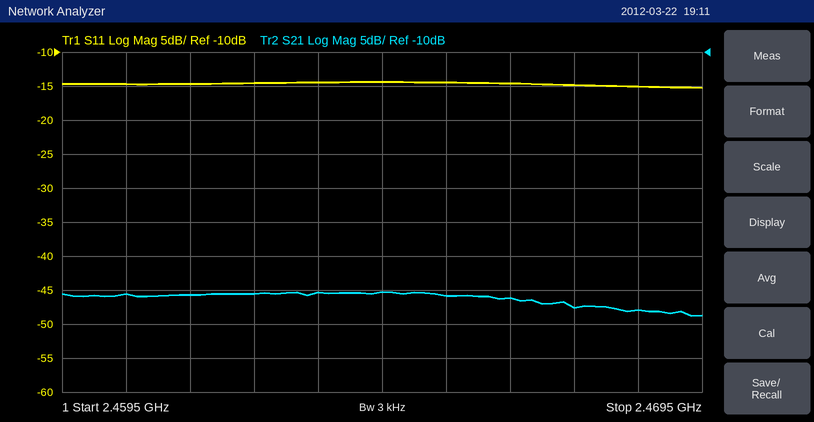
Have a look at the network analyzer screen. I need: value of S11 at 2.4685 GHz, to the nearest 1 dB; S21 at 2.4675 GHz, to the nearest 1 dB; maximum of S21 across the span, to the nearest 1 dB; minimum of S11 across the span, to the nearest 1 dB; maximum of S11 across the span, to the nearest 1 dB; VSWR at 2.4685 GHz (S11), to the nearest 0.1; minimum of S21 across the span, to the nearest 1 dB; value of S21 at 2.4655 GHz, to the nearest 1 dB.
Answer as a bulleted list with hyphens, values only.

- -15 dB
- -48 dB
- -45 dB
- -15 dB
- -14 dB
- 1.4
- -49 dB
- -46 dB
